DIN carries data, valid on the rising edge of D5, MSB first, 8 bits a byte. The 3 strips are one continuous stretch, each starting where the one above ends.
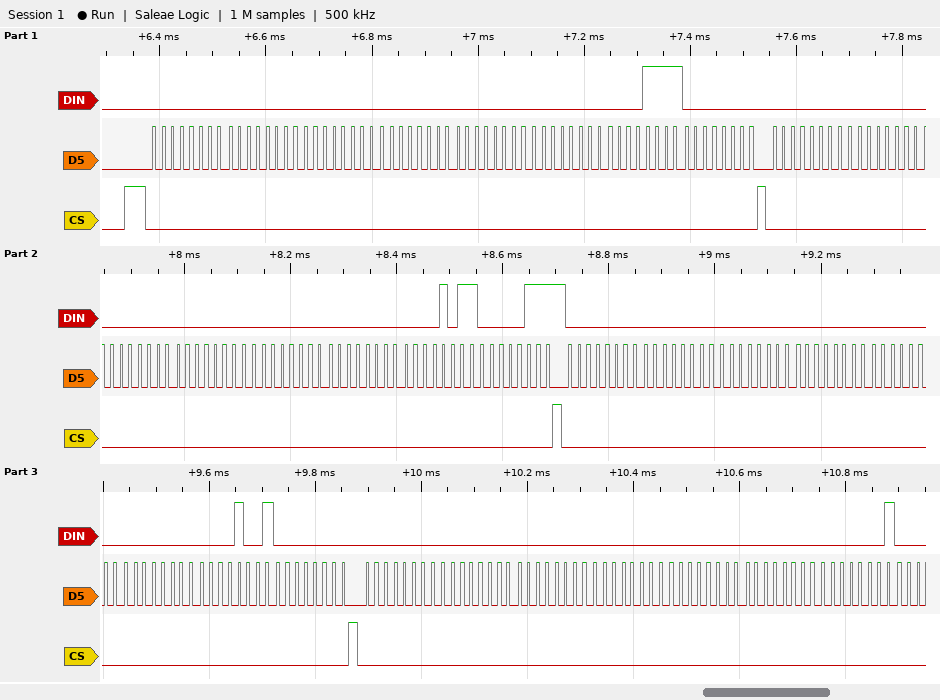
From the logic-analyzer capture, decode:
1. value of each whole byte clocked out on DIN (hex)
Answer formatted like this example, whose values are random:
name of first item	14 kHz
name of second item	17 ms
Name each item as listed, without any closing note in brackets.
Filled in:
value of each whole byte clocked out on DIN	00 00 00 00 00 00 0F 00 00 00 00 00 00 00 0B 07 00 00 00 00 00 00 09 00 00 00 00 00 00 00 01
